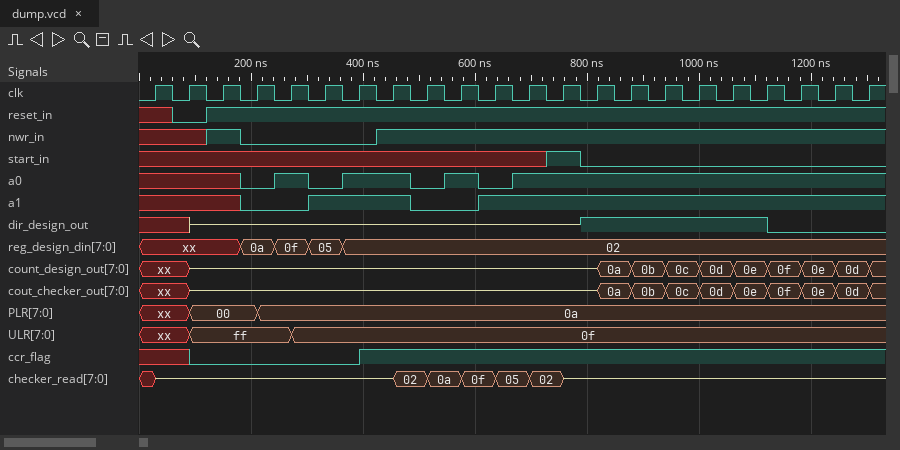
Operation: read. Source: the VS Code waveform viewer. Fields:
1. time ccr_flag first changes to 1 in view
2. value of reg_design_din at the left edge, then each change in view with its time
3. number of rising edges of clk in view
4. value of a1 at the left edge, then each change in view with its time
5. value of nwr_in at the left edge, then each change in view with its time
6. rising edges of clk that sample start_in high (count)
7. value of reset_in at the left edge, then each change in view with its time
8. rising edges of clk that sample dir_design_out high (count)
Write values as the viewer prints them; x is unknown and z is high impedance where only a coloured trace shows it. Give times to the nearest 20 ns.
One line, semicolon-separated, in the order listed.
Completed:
400 ns; xx, 0a at 180 ns, 0f at 240 ns, 05 at 300 ns, 02 at 360 ns; 22; x, 0 at 180 ns, 1 at 300 ns, 0 at 480 ns, 1 at 600 ns; x, 1 at 120 ns, 0 at 180 ns, 1 at 420 ns; 1; x, 0 at 60 ns, 1 at 120 ns; 6
